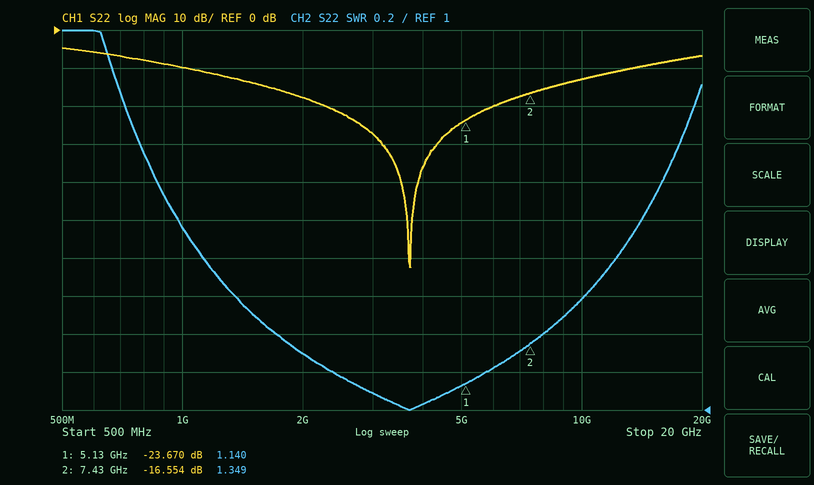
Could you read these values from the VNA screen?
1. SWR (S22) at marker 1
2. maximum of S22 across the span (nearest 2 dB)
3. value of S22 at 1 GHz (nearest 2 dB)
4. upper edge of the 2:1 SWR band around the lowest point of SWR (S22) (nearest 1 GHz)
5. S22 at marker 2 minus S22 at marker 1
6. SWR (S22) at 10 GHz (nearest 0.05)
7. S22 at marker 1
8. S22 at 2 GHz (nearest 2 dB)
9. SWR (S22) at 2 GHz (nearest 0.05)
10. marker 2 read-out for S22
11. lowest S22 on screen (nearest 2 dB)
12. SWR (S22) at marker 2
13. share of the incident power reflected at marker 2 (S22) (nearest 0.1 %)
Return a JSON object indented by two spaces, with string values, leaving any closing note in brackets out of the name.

{
  "SWR (S22) at marker 1": "1.140",
  "maximum of S22 across the span": "-4 dB",
  "value of S22 at 1 GHz": "-10 dB",
  "upper edge of the 2:1 SWR band around the lowest point of SWR (S22)": "14 GHz",
  "S22 at marker 2 minus S22 at marker 1": "7.116 dB",
  "SWR (S22) at 10 GHz": "1.60",
  "S22 at marker 1": "-23.670 dB",
  "S22 at 2 GHz": "-18 dB",
  "SWR (S22) at 2 GHz": "1.30",
  "marker 2 read-out for S22": "-16.554 dB",
  "lowest S22 on screen": "-62 dB",
  "SWR (S22) at marker 2": "1.349",
  "share of the incident power reflected at marker 2 (S22)": "2.2 %"
}
